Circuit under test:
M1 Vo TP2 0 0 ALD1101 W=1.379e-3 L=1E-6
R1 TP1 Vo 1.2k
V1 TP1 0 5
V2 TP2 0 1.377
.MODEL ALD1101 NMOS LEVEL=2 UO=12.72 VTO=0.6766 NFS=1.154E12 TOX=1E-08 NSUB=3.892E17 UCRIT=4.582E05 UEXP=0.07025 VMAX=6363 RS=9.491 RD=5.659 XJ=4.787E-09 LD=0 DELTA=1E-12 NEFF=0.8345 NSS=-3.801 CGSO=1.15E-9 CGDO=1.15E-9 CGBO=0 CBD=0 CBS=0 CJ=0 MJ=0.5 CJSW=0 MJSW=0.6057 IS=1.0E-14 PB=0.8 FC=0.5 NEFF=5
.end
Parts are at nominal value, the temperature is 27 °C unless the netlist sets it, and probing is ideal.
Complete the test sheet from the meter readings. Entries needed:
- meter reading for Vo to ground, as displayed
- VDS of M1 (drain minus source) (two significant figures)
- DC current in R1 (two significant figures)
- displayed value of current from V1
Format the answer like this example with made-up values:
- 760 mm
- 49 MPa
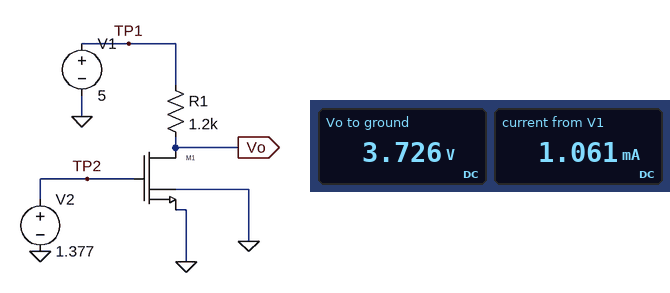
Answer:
- 3.726 V
- 3.7 V
- 1.1 mA
- 1.061 mA
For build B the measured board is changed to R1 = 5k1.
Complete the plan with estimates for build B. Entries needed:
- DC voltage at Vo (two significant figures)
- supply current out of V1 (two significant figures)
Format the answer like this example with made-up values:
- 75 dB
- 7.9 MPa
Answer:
- 340 mV
- 910 µA
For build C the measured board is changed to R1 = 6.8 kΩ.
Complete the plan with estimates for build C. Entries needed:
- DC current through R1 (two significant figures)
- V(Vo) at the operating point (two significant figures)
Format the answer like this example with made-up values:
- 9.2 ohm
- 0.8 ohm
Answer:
- 700 µA
- 220 mV
